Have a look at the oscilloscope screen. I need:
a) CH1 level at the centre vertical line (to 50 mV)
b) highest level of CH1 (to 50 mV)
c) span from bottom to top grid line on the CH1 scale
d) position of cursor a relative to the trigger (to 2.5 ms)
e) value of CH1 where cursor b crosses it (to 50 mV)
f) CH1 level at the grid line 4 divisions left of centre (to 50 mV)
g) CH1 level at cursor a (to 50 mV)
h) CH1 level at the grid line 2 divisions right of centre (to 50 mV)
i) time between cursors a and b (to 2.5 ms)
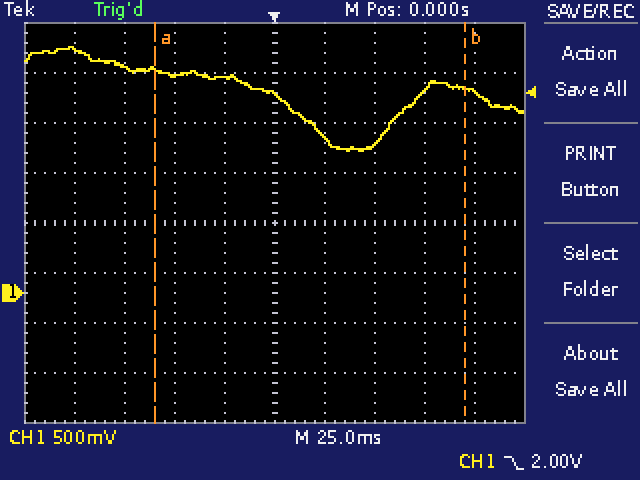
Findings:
2.00 V
2.45 V
4 V
-60.0 ms
2.05 V
2.45 V
2.25 V
1.50 V
155.0 ms
